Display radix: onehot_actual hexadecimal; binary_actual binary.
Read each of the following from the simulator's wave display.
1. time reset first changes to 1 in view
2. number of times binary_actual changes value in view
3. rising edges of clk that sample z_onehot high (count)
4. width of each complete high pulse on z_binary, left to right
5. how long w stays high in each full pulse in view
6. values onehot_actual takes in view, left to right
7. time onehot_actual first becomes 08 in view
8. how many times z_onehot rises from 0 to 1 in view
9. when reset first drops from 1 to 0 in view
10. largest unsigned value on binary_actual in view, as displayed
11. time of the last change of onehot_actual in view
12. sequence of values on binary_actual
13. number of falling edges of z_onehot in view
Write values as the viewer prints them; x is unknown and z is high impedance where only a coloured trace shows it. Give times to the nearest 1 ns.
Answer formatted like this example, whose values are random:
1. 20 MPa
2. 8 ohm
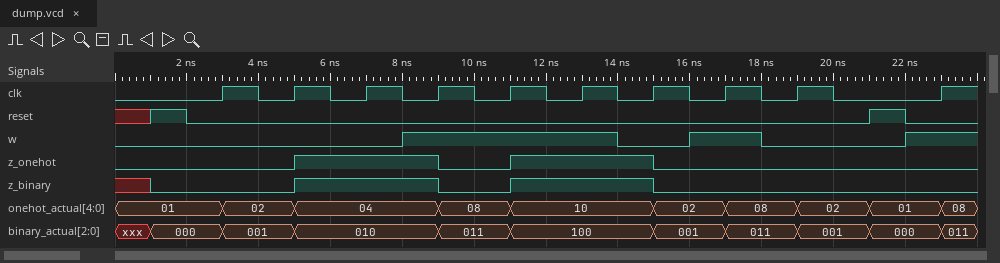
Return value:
1. 1 ns
2. 10
3. 4
4. 4 ns, 4 ns
5. 6 ns, 2 ns
6. 01, 02, 04, 08, 10, 02, 08, 02, 01, 08
7. 9 ns
8. 2
9. 2 ns
10. 100
11. 23 ns
12. xxx, 000, 001, 010, 011, 100, 001, 011, 001, 000, 011
13. 2
